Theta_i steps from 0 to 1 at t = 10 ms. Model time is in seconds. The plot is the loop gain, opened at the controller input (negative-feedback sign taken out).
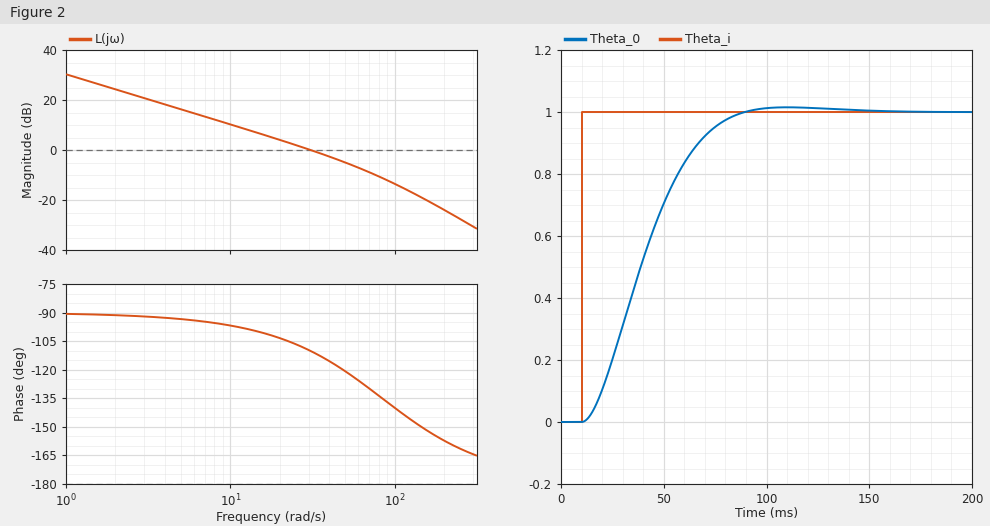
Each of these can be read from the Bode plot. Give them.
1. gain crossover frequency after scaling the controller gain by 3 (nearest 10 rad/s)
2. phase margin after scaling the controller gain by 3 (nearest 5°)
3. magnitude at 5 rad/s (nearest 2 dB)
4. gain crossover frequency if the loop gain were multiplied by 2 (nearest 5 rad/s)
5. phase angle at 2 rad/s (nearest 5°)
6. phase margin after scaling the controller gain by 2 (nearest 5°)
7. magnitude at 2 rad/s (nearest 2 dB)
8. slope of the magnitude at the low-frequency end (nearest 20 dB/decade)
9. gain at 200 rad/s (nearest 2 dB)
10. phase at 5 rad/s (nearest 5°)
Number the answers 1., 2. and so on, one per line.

1. 70 rad/s
2. 50°
3. 16 dB
4. 55 rad/s
5. -90°
6. 55°
7. 24 dB
8. -20 dB/decade
9. -24 dB
10. -95°
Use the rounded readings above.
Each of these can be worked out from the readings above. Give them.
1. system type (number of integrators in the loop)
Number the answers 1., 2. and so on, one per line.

1. 1
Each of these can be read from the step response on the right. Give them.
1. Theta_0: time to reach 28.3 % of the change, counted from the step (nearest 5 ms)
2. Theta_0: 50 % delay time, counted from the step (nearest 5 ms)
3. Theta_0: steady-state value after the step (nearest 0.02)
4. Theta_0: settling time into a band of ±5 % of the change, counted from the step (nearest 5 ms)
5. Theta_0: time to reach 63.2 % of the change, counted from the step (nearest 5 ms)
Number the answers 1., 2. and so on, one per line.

1. 20 ms
2. 30 ms
3. 1.00
4. 65 ms
5. 35 ms
